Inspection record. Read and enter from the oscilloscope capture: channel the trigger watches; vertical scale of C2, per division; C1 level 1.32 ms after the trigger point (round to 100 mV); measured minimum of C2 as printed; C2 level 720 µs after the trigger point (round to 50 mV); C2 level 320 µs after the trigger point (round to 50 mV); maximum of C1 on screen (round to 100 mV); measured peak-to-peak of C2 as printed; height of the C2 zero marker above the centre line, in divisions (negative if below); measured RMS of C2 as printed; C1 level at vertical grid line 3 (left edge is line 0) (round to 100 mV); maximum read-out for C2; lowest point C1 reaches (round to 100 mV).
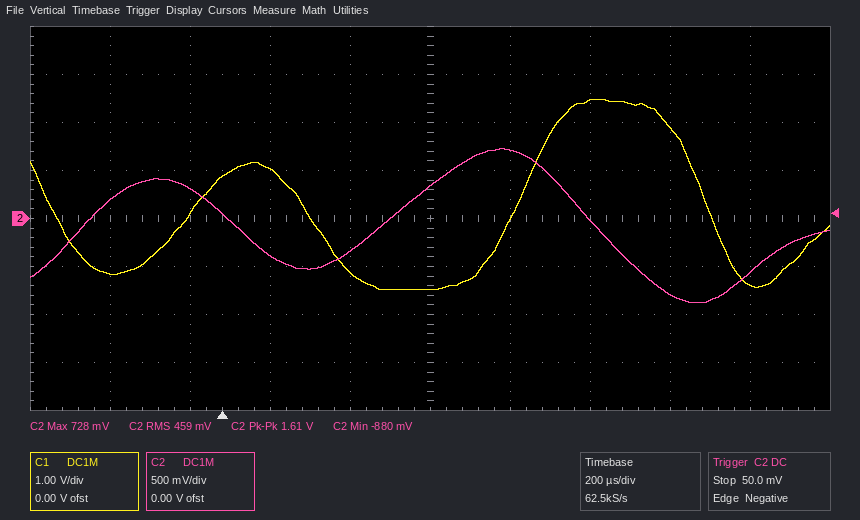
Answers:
C2
500 mV
-1.4 V
-880 mV
700 mV
-350 mV
2.5 V
1.61 V
0.0 div
459 mV
1.0 V
728 mV
-1.5 V
